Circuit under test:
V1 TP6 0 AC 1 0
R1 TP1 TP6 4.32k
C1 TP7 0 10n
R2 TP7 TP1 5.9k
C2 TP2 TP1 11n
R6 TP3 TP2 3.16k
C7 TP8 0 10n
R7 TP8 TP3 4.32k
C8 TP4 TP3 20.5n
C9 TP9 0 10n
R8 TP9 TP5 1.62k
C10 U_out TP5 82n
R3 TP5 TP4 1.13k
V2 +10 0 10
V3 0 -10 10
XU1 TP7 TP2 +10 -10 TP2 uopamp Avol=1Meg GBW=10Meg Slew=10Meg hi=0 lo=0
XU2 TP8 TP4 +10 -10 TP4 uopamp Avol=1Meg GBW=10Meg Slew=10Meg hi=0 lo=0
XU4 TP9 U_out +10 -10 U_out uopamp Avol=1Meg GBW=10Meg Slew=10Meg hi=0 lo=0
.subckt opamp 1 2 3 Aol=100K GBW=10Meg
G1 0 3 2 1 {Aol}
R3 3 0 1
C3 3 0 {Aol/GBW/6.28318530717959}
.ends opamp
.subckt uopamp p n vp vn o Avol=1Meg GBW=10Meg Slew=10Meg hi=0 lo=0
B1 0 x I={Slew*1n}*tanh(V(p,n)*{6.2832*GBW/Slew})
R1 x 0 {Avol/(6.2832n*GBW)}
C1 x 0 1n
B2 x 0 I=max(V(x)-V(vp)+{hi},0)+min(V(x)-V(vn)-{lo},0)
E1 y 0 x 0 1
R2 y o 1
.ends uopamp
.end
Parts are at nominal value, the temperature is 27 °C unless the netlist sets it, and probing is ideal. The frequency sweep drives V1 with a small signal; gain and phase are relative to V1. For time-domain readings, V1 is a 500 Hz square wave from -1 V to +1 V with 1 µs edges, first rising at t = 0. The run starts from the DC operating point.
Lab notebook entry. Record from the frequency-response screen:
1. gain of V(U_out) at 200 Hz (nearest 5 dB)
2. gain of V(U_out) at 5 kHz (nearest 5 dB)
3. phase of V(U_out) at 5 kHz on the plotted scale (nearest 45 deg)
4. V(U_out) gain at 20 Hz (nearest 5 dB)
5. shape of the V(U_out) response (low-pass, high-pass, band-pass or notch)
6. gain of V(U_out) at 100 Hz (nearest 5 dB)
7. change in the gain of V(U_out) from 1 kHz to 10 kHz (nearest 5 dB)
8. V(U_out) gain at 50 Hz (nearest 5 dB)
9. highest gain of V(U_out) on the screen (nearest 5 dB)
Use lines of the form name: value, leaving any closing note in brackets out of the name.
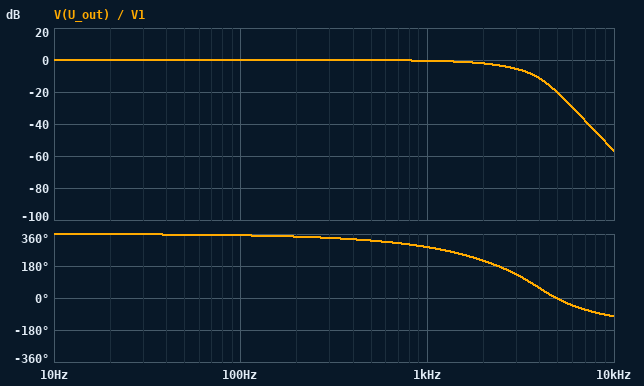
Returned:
gain of V(U_out) at 200 Hz: 0 dB
gain of V(U_out) at 5 kHz: -20 dB
phase of V(U_out) at 5 kHz on the plotted scale: 0 deg
V(U_out) gain at 20 Hz: 0 dB
shape of the V(U_out) response: low-pass
gain of V(U_out) at 100 Hz: 0 dB
change in the gain of V(U_out) from 1 kHz to 10 kHz: -55 dB
V(U_out) gain at 50 Hz: 0 dB
highest gain of V(U_out) on the screen: 0 dB
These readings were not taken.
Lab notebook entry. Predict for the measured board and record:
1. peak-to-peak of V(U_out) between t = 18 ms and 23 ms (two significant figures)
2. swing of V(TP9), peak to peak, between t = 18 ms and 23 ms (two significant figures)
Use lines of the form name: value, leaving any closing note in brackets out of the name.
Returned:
peak-to-peak of V(U_out) between t = 18 ms and 23 ms: 2.1 V
swing of V(TP9), peak to peak, between t = 18 ms and 23 ms: 2.1 V
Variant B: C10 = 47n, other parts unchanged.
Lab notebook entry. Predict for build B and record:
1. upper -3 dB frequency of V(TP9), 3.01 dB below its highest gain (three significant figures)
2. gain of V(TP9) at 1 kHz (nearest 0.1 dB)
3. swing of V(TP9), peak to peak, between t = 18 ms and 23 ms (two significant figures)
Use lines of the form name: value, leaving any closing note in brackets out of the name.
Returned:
upper -3 dB frequency of V(TP9), 3.01 dB below its highest gain: 1.98 kHz
gain of V(TP9) at 1 kHz: -0.7 dB
swing of V(TP9), peak to peak, between t = 18 ms and 23 ms: 2.0 V
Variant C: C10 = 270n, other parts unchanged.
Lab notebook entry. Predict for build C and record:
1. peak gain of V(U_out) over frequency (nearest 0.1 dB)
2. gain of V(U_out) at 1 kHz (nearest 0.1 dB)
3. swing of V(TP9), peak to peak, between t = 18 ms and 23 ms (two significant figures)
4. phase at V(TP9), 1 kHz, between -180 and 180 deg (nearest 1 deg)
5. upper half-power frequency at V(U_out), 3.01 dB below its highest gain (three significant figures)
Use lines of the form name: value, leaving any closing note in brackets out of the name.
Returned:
peak gain of V(U_out) over frequency: 4.1 dB
gain of V(U_out) at 1 kHz: 0.8 dB
swing of V(TP9), peak to peak, between t = 18 ms and 23 ms: 3.2 V
phase at V(TP9), 1 kHz, between -180 and 180 deg: -76 deg
upper half-power frequency at V(U_out), 3.01 dB below its highest gain: 2.45 kHz
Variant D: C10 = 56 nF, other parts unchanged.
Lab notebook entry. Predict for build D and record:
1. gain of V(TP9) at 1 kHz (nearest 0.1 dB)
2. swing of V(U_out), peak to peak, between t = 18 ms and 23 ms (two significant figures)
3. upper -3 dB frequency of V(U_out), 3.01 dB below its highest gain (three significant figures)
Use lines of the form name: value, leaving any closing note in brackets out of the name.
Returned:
gain of V(TP9) at 1 kHz: -0.6 dB
swing of V(U_out), peak to peak, between t = 18 ms and 23 ms: 2.0 V
upper -3 dB frequency of V(U_out), 3.01 dB below its highest gain: 2.05 kHz
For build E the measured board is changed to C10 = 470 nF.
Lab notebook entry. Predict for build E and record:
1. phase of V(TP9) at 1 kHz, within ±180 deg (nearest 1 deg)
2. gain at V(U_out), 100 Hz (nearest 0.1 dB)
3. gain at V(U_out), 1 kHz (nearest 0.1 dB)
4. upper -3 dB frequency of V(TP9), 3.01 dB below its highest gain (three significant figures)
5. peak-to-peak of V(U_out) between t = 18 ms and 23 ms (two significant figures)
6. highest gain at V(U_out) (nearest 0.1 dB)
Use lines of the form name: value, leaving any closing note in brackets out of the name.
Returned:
phase of V(TP9) at 1 kHz, within ±180 deg: -78 deg
gain at V(U_out), 100 Hz: 0 dB
gain at V(U_out), 1 kHz: 2.5 dB
upper -3 dB frequency of V(TP9), 3.01 dB below its highest gain: 1.88 kHz
peak-to-peak of V(U_out) between t = 18 ms and 23 ms: 4.0 V
highest gain at V(U_out): 8.2 dB
